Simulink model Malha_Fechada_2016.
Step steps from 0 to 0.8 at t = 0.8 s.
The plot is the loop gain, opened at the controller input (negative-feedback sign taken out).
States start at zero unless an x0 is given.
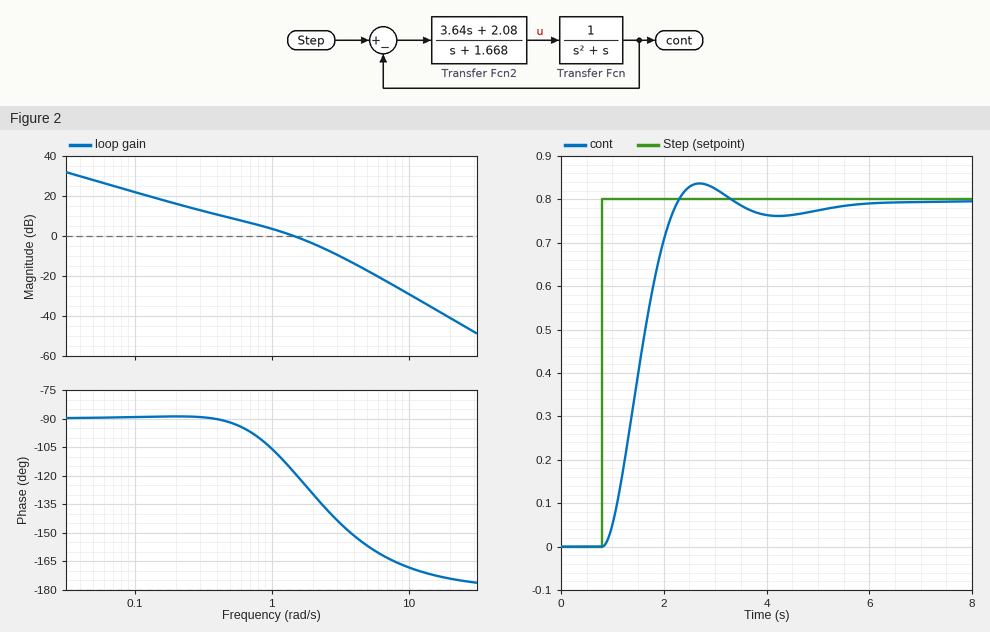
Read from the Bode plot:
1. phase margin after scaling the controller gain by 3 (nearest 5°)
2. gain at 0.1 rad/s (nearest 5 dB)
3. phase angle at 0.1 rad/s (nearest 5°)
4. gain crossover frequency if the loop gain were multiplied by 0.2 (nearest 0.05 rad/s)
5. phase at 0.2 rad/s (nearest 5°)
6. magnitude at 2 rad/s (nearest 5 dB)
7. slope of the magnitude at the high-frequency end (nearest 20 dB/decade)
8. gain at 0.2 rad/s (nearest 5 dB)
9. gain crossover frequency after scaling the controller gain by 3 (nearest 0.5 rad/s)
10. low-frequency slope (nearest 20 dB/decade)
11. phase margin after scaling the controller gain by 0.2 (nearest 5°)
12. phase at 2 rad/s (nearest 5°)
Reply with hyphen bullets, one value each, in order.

- 35°
- 20 dB
- -90°
- 0.25 rad/s
- -90°
- -5 dB
- -40 dB/decade
- 15 dB
- 3.0 rad/s
- -20 dB/decade
- 90°
- -130°
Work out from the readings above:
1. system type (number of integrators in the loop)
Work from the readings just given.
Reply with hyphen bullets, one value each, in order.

- 1
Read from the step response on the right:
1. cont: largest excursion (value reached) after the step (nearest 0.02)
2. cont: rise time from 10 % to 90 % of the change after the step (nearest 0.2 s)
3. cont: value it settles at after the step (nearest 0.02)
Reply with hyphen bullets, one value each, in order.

- 0.84
- 1.0 s
- 0.80
